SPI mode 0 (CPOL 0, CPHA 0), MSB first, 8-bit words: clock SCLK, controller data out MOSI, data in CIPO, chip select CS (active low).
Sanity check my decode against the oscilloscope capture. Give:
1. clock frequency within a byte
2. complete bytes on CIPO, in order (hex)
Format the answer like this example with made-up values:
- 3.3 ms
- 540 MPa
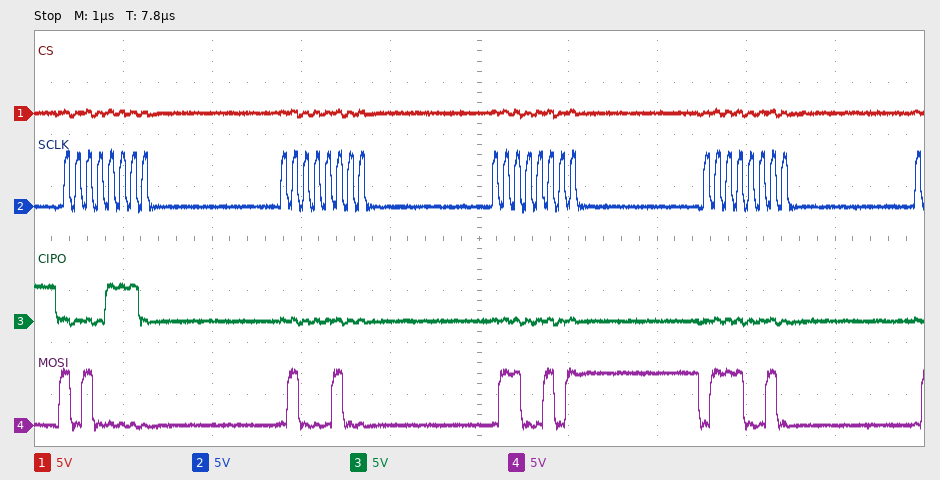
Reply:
- 8 MHz
- 0E 00 00 00
